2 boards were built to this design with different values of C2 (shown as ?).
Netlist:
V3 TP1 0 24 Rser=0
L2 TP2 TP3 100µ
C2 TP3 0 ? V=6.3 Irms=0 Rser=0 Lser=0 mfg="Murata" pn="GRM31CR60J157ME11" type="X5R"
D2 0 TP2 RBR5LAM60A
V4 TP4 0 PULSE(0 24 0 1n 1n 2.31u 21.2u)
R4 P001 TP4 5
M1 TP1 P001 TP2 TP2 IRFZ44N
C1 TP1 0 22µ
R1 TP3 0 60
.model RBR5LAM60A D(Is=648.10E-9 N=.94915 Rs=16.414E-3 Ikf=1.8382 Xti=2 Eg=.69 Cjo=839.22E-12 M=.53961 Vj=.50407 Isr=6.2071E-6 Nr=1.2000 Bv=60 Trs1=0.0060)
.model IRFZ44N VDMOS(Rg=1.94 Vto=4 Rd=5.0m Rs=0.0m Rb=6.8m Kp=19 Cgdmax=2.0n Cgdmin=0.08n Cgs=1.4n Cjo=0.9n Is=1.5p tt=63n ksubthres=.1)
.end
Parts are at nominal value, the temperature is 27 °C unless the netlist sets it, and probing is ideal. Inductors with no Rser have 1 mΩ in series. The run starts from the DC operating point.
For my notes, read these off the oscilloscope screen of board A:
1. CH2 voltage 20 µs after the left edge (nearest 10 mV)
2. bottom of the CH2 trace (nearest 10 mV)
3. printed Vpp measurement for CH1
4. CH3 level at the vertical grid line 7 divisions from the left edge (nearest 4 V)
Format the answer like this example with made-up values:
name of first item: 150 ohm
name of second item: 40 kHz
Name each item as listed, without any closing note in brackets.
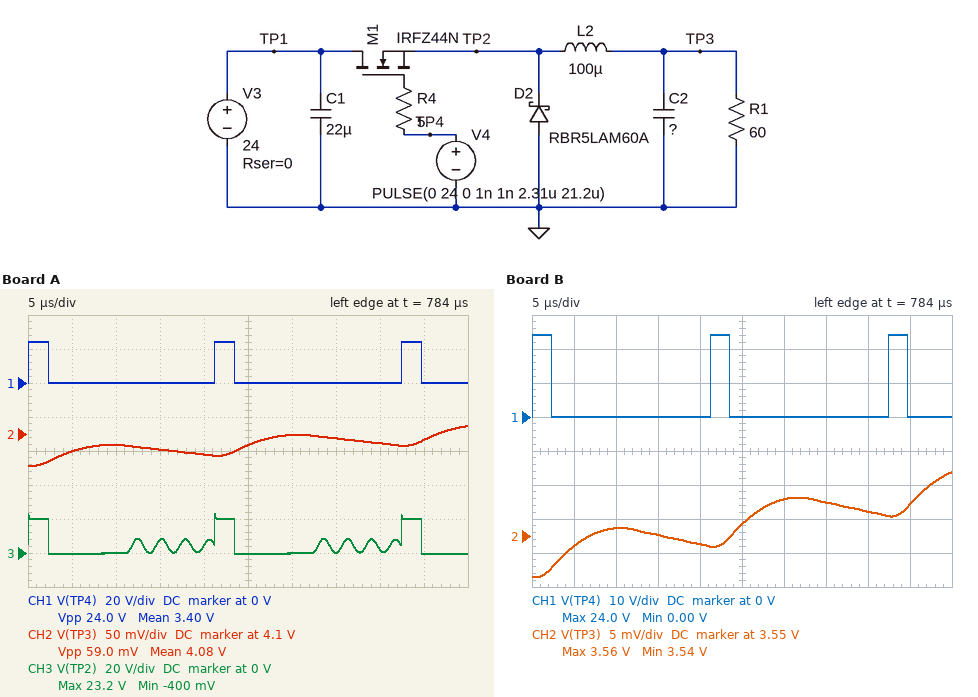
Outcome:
CH2 voltage 20 µs after the left edge: 4.07 V
bottom of the CH2 trace: 4.05 V
printed Vpp measurement for CH1: 24.0 V
CH3 level at the vertical grid line 7 divisions from the left edge: 0 V
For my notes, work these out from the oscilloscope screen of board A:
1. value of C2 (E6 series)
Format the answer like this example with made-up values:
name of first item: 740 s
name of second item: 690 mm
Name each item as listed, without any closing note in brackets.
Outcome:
value of C2: 47 µF
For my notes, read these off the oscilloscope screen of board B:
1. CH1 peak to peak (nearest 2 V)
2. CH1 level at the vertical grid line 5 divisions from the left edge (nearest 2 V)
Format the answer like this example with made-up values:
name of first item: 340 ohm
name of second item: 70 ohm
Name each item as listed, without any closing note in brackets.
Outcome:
CH1 peak to peak: 24 V
CH1 level at the vertical grid line 5 divisions from the left edge: 0 V
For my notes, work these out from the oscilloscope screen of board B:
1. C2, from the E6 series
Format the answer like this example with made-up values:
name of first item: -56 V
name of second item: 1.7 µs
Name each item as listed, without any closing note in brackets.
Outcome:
C2, from the E6 series: 220 µF
